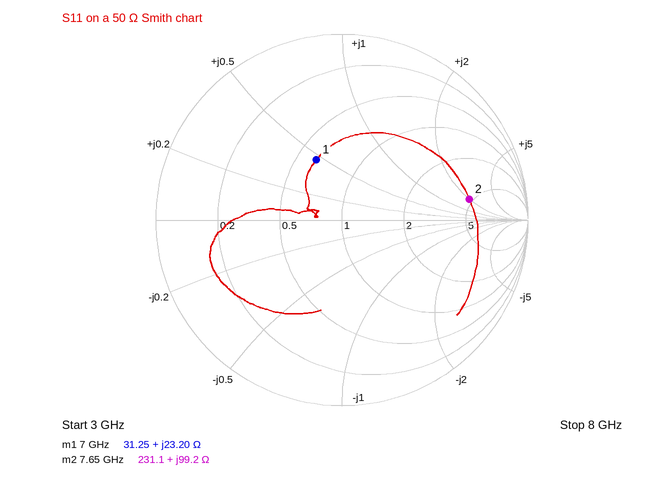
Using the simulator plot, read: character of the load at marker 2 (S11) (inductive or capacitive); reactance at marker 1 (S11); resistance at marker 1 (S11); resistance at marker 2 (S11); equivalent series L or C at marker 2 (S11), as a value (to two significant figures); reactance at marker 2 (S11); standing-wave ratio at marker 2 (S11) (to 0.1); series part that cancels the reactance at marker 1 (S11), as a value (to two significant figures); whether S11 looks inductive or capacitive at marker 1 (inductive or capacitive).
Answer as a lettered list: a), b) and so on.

a) inductive
b) +23.20 Ω
c) 31.25 Ω
d) 231.1 Ω
e) 2.1 nH
f) +99.2 Ω
g) 5.5
h) 980 fF
i) inductive
